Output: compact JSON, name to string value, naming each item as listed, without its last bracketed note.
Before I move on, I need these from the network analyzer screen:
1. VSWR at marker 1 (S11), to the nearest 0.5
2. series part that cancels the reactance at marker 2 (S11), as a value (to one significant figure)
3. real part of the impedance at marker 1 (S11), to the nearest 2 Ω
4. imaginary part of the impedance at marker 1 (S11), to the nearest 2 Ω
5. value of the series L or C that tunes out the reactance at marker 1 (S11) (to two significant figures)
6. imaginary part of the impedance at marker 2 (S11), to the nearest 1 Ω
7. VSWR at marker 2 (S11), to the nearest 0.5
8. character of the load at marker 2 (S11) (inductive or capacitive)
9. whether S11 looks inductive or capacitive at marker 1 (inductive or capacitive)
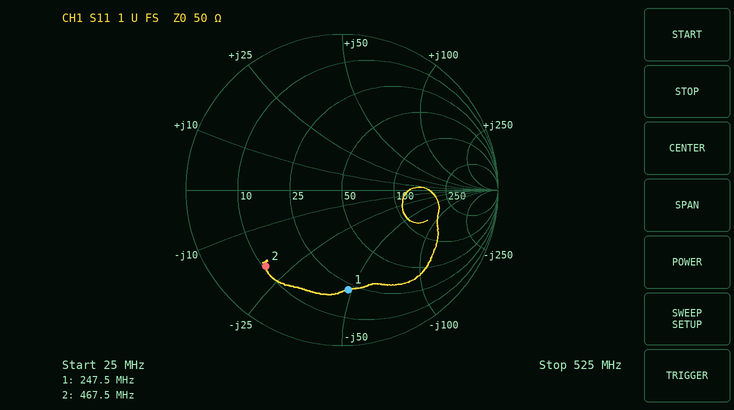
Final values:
{"VSWR at marker 1 (S11), to the nearest 0.5": "4.5", "series part that cancels the reactance at marker 2 (S11), as a value": "7 nH", "real part of the impedance at marker 1 (S11), to the nearest 2 Ω": "22 Ω", "imaginary part of the impedance at marker 1 (S11), to the nearest 2 Ω": "-48 Ω", "value of the series L or C that tunes out the reactance at marker 1 (S11)": "31 nH", "imaginary part of the impedance at marker 2 (S11), to the nearest 1 Ω": "-20 Ω", "VSWR at marker 2 (S11), to the nearest 0.5": "5.5", "character of the load at marker 2 (S11)": "capacitive", "whether S11 looks inductive or capacitive at marker 1": "capacitive"}
